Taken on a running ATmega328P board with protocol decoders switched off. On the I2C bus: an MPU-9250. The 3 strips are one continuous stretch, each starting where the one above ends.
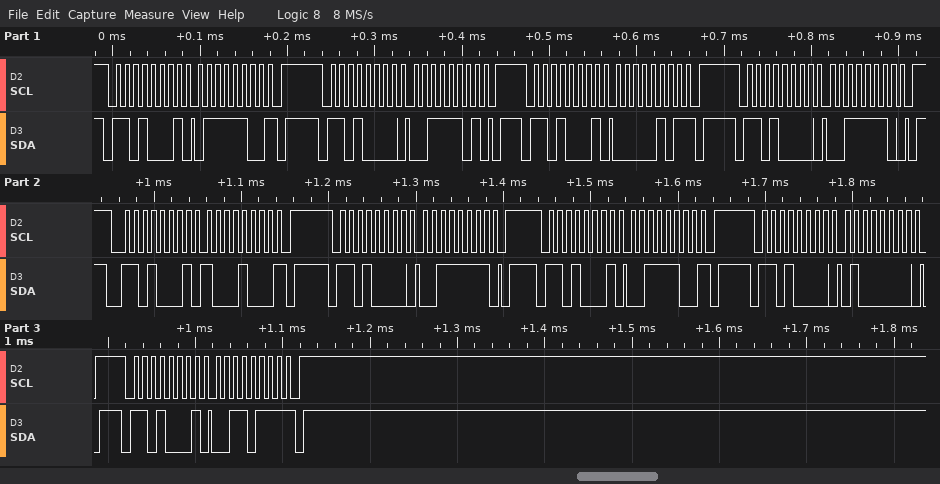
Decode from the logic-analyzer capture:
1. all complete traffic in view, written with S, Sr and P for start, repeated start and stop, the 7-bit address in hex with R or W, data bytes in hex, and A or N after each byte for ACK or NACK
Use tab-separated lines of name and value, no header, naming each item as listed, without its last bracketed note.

all complete traffic in view, written with S, Sr and P for start, repeated start and stop, the 7-bit address in hex with R or W, data bytes in hex, and A or N after each byte for ACK or NACK	S 68R A 7C N P S 68W A 3D A P S 68R A 05 N P S 68W A 3E A P S 68R A 88 N P S 68W A 3F A P S 68R A 3C N P S 68W A 40 A P S 68R A 37 N P
